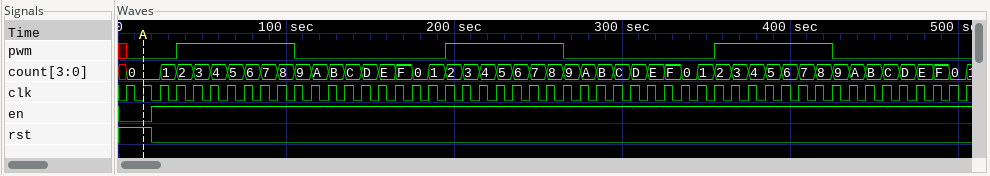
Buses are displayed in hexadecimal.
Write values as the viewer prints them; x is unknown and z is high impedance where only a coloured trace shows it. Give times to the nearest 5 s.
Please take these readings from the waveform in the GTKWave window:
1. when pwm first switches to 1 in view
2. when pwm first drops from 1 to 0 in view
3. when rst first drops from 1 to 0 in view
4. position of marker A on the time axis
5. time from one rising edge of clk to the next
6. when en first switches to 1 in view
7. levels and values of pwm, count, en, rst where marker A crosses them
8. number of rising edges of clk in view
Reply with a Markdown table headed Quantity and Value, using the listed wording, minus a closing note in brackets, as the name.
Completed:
| Quantity | Value |
|---|---|
| when pwm first switches to 1 in view | 35 s |
| when pwm first drops from 1 to 0 in view | 105 s |
| when rst first drops from 1 to 0 in view | 20 s |
| position of marker A on the time axis | 15 s |
| time from one rising edge of clk to the next | 10 s |
| when en first switches to 1 in view | 20 s |
| levels and values of pwm, count, en, rst where marker A crosses them | pwm=0, count=0, en=0, rst=1 |
| number of rising edges of clk in view | 51 |
